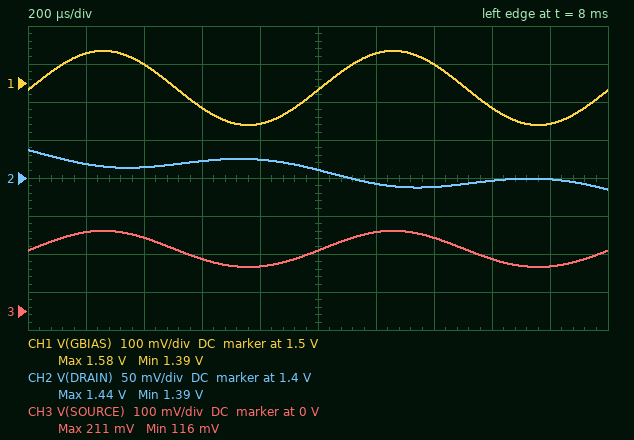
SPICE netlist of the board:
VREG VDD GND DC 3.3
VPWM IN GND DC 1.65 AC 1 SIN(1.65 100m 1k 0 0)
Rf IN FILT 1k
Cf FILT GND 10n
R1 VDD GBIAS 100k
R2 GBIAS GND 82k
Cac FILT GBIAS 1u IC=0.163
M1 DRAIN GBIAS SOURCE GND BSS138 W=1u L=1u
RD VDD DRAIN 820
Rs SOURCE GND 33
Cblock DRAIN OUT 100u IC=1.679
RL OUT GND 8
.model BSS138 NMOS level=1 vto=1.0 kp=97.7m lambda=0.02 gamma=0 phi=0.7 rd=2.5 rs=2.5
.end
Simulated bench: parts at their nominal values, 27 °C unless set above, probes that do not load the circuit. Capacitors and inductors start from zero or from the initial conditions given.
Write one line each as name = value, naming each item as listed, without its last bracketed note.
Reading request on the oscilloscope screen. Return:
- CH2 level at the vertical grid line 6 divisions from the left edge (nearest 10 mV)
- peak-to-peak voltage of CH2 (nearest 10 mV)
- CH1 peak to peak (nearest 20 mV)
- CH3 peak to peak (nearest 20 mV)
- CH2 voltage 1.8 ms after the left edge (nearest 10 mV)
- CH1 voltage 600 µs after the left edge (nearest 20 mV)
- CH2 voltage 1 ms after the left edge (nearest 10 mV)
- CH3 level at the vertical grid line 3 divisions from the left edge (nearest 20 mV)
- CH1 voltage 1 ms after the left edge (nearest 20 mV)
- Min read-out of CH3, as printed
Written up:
CH2 level at the vertical grid line 6 divisions from the left edge = 1.39 V
peak-to-peak voltage of CH2 = 50 mV
CH1 peak to peak = 200 mV
CH3 peak to peak = 100 mV
CH2 voltage 1.8 ms after the left edge = 1.40 V
CH1 voltage 600 µs after the left edge = 1.44 V
CH2 voltage 1 ms after the left edge = 1.41 V
CH3 level at the vertical grid line 3 divisions from the left edge = 140 mV
CH1 voltage 1 ms after the left edge = 1.48 V
Min read-out of CH3, as printed = 116 mV
